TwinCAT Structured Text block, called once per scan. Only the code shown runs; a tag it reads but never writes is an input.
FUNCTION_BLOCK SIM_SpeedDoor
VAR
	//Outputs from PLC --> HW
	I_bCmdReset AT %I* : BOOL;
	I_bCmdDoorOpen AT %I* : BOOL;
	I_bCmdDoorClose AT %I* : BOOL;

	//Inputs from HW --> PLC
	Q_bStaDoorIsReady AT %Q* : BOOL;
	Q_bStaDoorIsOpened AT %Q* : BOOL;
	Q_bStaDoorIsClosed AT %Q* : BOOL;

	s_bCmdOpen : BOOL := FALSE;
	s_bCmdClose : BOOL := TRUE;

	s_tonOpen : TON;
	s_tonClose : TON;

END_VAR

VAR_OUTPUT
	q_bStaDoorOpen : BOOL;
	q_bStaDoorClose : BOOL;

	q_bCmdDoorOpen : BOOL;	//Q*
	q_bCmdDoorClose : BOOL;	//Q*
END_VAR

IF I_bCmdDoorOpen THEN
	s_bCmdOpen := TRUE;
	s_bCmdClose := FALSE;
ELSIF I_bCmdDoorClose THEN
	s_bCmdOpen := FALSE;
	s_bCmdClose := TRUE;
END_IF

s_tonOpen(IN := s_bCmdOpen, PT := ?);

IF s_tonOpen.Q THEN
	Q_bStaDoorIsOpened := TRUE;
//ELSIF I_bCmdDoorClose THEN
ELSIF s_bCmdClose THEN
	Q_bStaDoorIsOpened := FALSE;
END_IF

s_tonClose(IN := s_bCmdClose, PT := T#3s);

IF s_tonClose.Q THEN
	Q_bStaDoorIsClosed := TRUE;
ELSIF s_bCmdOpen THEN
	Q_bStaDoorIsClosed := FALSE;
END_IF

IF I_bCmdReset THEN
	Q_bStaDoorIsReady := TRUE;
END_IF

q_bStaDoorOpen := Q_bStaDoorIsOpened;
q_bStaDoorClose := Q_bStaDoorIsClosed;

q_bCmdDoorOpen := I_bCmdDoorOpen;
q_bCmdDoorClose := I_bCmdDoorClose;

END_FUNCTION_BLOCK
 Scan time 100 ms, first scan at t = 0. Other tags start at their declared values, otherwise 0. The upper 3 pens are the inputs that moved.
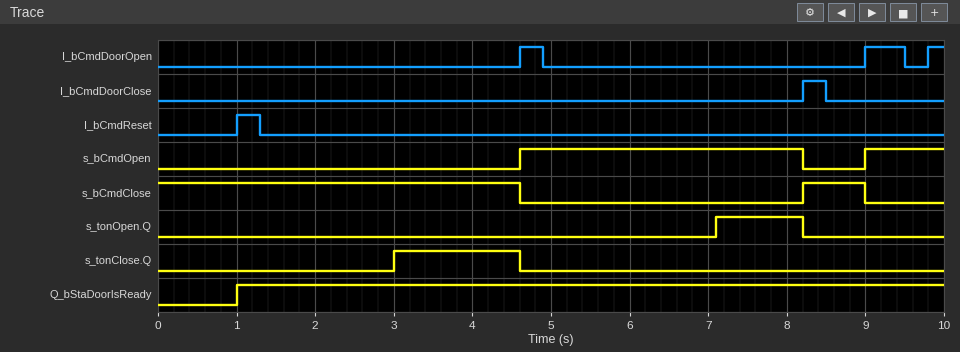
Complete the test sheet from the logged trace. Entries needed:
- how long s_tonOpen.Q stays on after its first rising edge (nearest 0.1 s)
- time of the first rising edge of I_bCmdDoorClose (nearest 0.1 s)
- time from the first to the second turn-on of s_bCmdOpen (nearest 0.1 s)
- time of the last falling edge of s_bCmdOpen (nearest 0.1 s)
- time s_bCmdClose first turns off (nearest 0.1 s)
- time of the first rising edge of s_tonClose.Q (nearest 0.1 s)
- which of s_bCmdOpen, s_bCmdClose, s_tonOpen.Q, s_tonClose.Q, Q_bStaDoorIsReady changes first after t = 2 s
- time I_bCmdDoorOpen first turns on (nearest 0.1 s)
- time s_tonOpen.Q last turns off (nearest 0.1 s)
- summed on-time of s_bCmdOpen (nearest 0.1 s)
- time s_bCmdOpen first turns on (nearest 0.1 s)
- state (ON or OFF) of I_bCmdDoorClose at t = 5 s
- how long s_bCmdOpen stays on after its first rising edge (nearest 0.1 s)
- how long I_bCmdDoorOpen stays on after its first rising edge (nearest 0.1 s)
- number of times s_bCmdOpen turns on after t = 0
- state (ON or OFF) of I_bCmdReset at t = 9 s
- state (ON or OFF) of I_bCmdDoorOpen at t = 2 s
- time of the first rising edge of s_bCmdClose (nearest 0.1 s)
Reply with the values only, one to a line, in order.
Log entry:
1.1 s
8.2 s
4.4 s
8.2 s
4.6 s
3.0 s
s_tonClose.Q
4.6 s
8.2 s
4.6 s
4.6 s
OFF
3.6 s
0.3 s
2
OFF
OFF
8.2 s
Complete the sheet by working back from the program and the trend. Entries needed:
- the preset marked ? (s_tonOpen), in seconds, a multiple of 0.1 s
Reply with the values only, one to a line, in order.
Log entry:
2.5 s
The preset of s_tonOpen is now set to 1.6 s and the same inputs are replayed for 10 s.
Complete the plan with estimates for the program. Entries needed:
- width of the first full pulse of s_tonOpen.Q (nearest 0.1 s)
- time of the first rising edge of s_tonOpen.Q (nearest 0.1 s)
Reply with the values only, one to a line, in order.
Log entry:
2.0 s
6.2 s
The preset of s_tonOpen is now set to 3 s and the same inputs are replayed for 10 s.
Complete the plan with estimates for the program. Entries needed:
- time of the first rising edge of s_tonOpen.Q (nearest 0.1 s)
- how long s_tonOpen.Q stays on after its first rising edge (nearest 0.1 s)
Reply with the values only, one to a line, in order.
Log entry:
7.6 s
0.6 s
